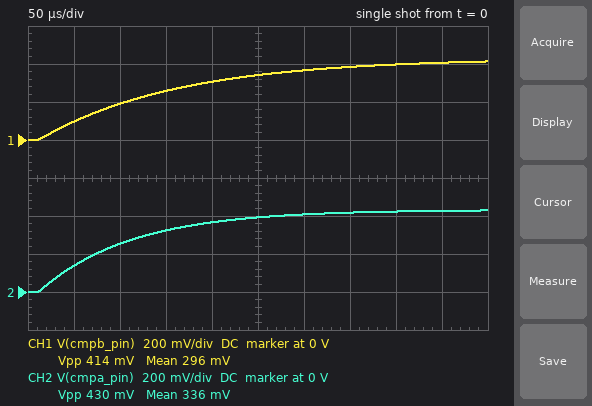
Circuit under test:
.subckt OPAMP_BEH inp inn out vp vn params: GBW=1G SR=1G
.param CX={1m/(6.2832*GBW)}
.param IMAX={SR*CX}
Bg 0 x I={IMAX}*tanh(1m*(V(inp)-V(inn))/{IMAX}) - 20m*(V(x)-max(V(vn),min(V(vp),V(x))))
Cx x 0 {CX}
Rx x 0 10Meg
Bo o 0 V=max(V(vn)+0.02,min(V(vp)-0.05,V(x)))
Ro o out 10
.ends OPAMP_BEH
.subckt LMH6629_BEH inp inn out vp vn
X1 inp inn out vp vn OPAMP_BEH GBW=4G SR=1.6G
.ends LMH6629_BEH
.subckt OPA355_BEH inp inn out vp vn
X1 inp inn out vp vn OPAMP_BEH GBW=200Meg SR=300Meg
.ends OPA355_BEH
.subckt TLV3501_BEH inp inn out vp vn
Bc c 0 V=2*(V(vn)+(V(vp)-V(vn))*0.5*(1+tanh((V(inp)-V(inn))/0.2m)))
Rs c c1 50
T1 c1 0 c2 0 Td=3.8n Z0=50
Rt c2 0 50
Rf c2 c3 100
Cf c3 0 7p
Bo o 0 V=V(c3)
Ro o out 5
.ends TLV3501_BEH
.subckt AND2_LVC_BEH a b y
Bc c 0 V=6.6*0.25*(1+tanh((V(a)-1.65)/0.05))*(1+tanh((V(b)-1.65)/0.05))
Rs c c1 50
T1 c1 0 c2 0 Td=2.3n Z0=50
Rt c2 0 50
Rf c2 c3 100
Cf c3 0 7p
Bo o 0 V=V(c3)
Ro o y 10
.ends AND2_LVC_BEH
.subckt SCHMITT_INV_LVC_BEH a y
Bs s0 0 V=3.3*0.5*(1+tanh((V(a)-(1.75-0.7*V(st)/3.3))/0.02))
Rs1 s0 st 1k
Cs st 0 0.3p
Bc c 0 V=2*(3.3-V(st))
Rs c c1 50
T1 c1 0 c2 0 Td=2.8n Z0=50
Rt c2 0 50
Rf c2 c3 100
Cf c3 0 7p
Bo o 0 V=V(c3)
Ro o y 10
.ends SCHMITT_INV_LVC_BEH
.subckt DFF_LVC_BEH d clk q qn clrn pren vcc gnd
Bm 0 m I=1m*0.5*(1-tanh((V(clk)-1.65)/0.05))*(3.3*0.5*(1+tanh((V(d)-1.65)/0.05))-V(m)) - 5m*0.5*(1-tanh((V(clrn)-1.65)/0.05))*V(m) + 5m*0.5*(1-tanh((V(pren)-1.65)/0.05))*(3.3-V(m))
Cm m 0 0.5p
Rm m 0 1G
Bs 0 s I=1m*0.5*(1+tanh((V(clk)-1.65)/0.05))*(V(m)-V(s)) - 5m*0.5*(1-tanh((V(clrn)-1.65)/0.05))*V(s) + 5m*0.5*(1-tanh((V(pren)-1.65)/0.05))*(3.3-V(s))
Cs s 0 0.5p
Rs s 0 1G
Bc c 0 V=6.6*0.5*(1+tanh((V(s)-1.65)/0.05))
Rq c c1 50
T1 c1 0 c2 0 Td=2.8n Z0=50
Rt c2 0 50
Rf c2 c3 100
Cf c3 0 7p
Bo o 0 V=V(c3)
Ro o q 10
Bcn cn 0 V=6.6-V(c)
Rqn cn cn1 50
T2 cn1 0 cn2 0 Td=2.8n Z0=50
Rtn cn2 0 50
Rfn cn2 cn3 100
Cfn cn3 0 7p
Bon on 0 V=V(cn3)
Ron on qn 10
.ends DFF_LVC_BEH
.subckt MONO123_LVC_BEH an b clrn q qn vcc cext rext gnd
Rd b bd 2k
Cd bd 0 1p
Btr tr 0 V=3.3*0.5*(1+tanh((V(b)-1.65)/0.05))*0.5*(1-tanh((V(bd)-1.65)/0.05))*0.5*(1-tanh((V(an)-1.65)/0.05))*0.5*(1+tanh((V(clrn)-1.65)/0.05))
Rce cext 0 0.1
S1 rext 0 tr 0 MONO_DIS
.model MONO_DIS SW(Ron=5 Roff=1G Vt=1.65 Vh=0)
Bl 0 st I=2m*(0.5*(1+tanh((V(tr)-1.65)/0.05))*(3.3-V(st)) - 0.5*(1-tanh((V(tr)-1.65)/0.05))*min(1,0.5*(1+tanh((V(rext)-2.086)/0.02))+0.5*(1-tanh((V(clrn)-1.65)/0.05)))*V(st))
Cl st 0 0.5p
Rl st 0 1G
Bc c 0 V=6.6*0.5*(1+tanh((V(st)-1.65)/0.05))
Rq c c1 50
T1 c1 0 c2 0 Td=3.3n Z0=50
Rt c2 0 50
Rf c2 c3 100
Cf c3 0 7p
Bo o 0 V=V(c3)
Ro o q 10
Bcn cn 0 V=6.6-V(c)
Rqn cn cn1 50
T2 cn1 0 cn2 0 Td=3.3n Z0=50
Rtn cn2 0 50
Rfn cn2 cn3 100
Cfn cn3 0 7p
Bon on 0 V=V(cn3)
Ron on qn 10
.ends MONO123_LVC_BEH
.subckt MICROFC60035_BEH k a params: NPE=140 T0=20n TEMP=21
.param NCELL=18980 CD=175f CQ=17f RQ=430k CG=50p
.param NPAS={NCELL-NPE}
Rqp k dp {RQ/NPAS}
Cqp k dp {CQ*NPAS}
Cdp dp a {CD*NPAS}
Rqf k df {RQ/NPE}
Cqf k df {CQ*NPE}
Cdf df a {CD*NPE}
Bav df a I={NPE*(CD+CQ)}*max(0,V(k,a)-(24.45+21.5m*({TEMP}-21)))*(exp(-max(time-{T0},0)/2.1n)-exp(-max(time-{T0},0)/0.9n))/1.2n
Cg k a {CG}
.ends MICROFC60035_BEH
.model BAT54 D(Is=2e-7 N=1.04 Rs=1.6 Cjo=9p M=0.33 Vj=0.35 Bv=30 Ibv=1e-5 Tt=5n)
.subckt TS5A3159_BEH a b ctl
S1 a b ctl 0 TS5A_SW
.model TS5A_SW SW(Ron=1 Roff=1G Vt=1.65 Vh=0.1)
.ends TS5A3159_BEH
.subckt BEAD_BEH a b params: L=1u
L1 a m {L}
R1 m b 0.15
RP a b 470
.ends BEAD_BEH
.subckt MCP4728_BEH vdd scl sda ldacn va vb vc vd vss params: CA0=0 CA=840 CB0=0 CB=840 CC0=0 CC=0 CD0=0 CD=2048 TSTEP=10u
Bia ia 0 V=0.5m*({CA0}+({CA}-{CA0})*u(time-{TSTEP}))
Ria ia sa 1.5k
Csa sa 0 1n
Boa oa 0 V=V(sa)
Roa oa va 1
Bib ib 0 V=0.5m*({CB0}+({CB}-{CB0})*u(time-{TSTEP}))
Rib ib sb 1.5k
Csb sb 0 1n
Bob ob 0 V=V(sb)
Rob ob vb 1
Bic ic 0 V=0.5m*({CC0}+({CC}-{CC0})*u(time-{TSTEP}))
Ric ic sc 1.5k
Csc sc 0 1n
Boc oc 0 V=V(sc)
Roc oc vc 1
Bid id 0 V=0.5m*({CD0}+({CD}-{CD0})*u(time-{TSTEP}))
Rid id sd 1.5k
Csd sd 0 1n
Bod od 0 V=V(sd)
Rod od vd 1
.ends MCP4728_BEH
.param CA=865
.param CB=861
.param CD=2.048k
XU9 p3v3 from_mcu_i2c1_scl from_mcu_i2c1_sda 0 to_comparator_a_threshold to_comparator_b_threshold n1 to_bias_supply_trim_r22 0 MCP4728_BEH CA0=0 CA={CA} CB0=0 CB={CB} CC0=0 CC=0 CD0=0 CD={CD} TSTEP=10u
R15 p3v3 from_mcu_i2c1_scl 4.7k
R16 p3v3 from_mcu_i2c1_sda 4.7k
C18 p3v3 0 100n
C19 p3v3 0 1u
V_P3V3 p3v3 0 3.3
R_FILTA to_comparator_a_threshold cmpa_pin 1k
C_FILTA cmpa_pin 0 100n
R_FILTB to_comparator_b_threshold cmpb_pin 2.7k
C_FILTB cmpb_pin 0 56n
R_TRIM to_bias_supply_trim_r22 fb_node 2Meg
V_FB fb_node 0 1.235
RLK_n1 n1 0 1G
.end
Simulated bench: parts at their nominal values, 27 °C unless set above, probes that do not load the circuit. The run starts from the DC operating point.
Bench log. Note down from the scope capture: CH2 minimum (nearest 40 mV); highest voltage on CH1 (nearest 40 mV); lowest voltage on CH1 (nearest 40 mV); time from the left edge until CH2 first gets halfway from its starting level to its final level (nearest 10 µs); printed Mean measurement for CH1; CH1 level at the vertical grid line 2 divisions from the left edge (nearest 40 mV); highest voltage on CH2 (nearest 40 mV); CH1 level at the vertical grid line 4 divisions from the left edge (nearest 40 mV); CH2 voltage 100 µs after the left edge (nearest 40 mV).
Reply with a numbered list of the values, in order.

1. 0 V
2. 400 mV
3. 0 V
4. 80 µs
5. 296 mV
6. 200 mV
7. 440 mV
8. 320 mV
9. 240 mV
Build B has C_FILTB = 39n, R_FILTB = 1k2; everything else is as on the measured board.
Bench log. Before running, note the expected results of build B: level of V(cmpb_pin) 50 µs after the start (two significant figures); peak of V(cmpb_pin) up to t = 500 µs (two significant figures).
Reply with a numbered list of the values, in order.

1. 240 mV
2. 430 mV
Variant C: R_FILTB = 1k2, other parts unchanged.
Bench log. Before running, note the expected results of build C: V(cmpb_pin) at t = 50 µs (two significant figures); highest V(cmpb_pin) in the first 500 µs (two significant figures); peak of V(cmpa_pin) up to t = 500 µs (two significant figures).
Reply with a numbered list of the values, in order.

1. 190 mV
2. 430 mV
3. 430 mV
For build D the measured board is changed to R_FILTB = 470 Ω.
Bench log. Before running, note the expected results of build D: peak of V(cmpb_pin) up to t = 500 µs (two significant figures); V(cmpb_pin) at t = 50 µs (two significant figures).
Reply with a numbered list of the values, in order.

1. 430 mV
2. 330 mV
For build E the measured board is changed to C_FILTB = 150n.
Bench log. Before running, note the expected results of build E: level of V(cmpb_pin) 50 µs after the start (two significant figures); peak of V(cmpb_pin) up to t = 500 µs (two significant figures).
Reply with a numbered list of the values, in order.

1. 39 mV
2. 300 mV
